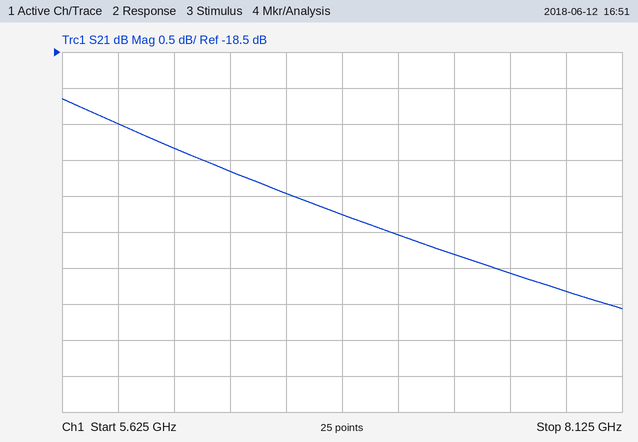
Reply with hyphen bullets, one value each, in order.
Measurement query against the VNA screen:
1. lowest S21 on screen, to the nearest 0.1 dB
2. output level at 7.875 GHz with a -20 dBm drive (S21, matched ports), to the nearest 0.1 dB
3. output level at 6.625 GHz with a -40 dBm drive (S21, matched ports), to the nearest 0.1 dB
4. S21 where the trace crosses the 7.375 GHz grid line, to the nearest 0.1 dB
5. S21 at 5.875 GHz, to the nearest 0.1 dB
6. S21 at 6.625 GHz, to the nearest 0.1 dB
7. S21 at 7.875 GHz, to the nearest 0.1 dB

- -22.1 dB
- -41.8 dBm
- -60.5 dBm
- -21.3 dB
- -19.5 dB
- -20.5 dB
- -21.8 dB
